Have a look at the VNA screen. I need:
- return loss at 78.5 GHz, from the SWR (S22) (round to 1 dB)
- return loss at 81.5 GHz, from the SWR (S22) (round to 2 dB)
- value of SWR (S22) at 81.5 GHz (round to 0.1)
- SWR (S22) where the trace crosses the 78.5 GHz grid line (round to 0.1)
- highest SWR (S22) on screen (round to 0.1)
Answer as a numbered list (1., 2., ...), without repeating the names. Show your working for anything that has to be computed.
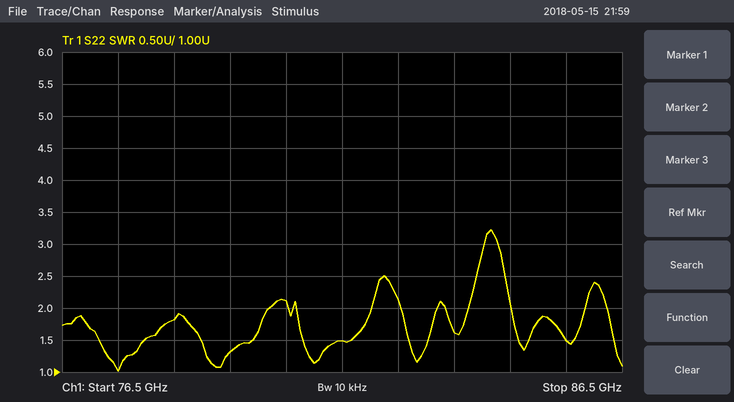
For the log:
1. −20 log10((1.8 − 1)/(1.8 + 1)) ≈ 11 dB
2. −20 log10((1.5 − 1)/(1.5 + 1)) ≈ 14 dB
3. 1.5
4. 1.8
5. 3.2
